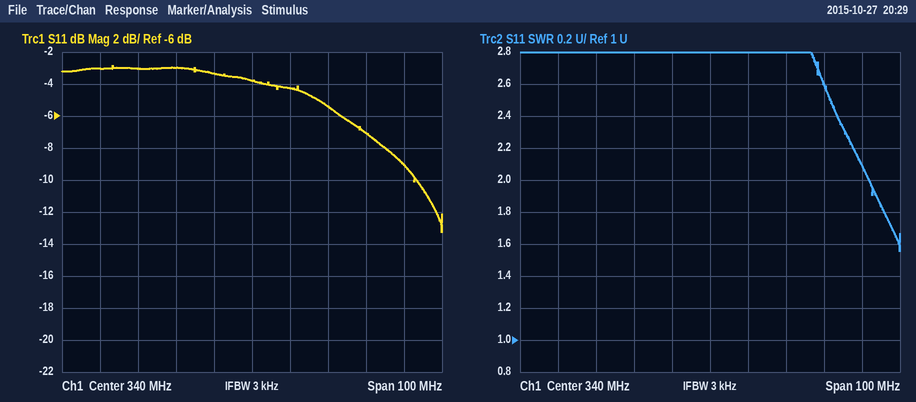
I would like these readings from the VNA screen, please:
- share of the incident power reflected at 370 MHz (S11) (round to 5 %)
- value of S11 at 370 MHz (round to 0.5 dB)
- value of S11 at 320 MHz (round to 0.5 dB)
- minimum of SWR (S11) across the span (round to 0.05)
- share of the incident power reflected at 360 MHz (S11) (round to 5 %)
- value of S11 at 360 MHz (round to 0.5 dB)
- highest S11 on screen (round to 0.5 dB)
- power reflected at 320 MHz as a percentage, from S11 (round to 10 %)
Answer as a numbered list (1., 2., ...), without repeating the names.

1. 20 %
2. -7.0 dB
3. -3.0 dB
4. 1.55
5. 30 %
6. -5.5 dB
7. -3.0 dB
8. 50 %
